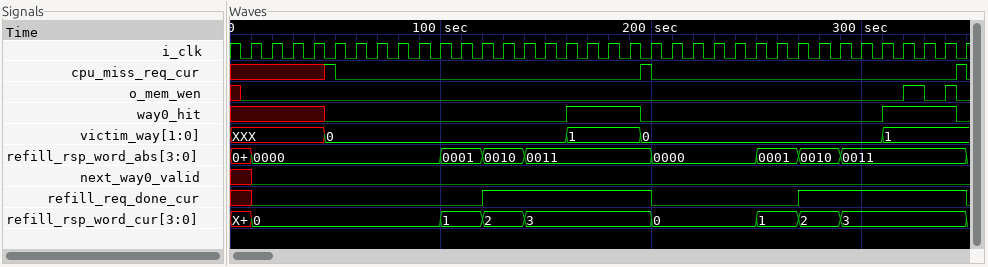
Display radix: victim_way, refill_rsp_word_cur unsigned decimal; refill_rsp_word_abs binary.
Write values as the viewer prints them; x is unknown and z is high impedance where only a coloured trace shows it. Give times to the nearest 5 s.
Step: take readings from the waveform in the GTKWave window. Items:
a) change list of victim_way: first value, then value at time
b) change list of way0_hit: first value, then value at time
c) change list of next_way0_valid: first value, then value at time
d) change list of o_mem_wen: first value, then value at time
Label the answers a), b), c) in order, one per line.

a) XXX, 0 at 45 s, 1 at 160 s, 0 at 195 s, 1 at 310 s
b) x, 0 at 45 s, 1 at 160 s, 0 at 195 s, 1 at 310 s, 0 at 345 s
c) x, 0 at 10 s
d) x, 0 at 5 s, 1 at 320 s, 0 at 330 s, 1 at 340 s, 0 at 345 s
